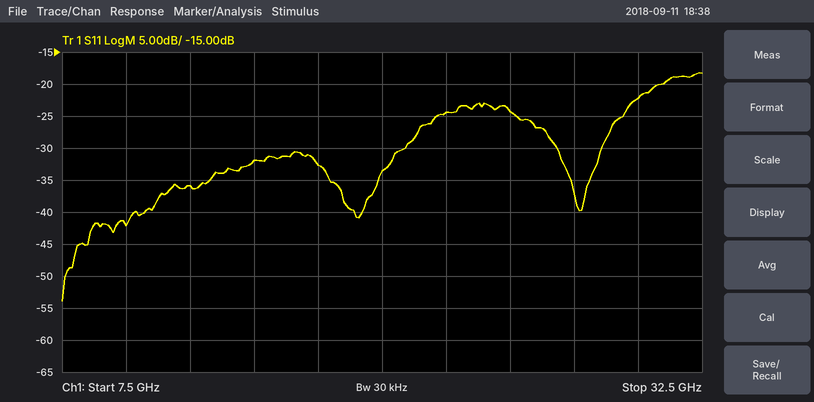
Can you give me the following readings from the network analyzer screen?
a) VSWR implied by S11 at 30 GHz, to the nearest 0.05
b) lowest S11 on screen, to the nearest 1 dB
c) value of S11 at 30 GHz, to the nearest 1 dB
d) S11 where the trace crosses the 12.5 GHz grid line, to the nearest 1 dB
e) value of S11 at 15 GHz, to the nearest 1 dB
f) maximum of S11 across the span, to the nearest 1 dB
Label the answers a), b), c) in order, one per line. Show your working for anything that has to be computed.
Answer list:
a) |Γ| = 10^(-22/20) = 0.0794; VSWR = (1 + 0.0794)/(1 − 0.0794) ≈ 1.17, so 1.15 to the nearest 0.05
b) -54 dB
c) -22 dB
d) -36 dB
e) -32 dB
f) -18 dB
